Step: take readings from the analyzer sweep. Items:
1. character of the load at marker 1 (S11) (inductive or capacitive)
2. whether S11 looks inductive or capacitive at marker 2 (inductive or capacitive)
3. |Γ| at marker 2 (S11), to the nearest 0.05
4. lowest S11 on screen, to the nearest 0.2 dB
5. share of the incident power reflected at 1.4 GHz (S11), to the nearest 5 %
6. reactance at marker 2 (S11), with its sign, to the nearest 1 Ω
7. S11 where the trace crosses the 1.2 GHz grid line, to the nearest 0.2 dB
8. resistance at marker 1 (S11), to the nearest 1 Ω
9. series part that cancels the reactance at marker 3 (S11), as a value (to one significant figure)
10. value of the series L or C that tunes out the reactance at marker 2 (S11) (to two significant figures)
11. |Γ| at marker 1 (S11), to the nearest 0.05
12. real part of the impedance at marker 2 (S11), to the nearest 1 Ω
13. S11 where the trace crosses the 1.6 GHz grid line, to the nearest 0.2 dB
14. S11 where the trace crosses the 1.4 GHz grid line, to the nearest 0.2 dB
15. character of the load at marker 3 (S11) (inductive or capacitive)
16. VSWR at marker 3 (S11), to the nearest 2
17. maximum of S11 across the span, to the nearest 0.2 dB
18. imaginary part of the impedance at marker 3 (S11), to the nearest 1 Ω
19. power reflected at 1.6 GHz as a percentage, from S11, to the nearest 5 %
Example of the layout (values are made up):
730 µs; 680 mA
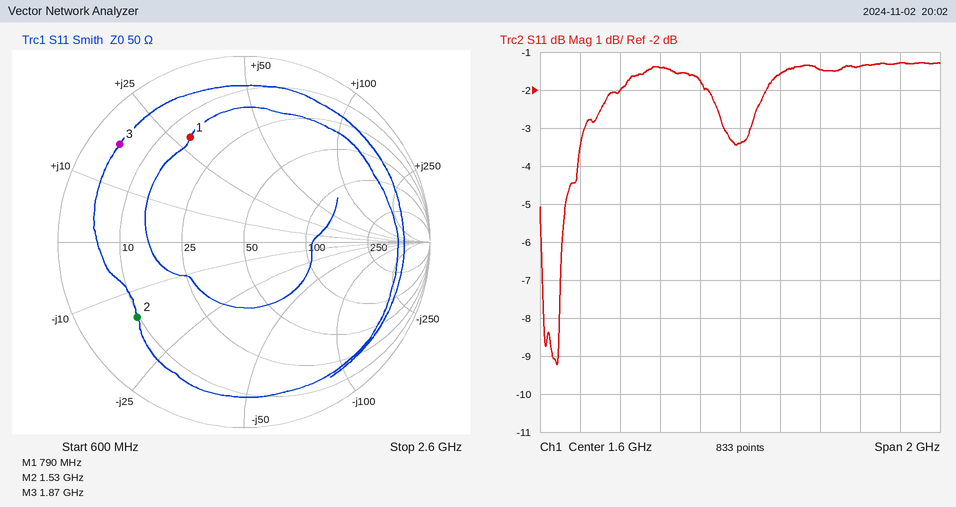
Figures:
inductive; capacitive; 0.70; -9.2 dB; 65 %; -15 Ω; -1.4 dB; 15 Ω; 5 pF; 1.6 nH; 0.65; 10 Ω; -3.4 dB; -1.8 dB; inductive; 12; -1.2 dB; +17 Ω; 45 %
